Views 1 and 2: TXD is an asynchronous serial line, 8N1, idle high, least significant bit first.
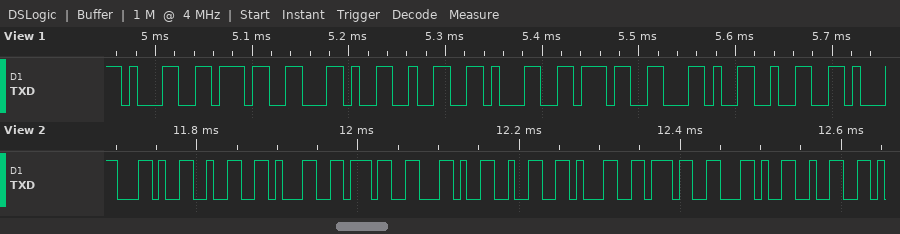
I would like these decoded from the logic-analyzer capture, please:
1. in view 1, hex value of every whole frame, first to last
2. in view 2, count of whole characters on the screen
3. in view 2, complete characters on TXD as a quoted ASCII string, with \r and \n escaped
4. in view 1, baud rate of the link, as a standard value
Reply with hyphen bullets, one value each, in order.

- 0x31 0x37 0x2C 0x32 0x31 0x37 0x2C 0x32
- 10
- ",217,217,2"
- 115200 baud
